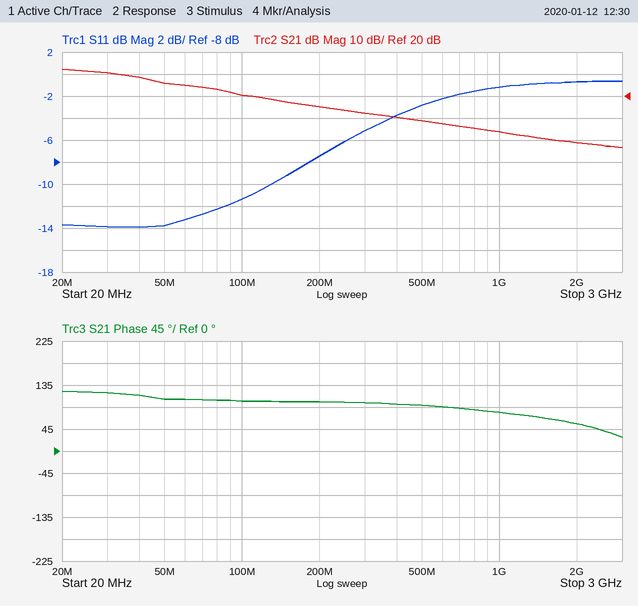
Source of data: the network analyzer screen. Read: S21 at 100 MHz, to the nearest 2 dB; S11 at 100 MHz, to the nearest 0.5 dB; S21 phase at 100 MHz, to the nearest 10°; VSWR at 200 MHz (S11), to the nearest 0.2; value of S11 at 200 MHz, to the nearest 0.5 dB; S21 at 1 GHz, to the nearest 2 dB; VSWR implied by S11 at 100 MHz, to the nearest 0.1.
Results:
20 dB
-11.5 dB
100°
2.4
-7.5 dB
4 dB
1.7
